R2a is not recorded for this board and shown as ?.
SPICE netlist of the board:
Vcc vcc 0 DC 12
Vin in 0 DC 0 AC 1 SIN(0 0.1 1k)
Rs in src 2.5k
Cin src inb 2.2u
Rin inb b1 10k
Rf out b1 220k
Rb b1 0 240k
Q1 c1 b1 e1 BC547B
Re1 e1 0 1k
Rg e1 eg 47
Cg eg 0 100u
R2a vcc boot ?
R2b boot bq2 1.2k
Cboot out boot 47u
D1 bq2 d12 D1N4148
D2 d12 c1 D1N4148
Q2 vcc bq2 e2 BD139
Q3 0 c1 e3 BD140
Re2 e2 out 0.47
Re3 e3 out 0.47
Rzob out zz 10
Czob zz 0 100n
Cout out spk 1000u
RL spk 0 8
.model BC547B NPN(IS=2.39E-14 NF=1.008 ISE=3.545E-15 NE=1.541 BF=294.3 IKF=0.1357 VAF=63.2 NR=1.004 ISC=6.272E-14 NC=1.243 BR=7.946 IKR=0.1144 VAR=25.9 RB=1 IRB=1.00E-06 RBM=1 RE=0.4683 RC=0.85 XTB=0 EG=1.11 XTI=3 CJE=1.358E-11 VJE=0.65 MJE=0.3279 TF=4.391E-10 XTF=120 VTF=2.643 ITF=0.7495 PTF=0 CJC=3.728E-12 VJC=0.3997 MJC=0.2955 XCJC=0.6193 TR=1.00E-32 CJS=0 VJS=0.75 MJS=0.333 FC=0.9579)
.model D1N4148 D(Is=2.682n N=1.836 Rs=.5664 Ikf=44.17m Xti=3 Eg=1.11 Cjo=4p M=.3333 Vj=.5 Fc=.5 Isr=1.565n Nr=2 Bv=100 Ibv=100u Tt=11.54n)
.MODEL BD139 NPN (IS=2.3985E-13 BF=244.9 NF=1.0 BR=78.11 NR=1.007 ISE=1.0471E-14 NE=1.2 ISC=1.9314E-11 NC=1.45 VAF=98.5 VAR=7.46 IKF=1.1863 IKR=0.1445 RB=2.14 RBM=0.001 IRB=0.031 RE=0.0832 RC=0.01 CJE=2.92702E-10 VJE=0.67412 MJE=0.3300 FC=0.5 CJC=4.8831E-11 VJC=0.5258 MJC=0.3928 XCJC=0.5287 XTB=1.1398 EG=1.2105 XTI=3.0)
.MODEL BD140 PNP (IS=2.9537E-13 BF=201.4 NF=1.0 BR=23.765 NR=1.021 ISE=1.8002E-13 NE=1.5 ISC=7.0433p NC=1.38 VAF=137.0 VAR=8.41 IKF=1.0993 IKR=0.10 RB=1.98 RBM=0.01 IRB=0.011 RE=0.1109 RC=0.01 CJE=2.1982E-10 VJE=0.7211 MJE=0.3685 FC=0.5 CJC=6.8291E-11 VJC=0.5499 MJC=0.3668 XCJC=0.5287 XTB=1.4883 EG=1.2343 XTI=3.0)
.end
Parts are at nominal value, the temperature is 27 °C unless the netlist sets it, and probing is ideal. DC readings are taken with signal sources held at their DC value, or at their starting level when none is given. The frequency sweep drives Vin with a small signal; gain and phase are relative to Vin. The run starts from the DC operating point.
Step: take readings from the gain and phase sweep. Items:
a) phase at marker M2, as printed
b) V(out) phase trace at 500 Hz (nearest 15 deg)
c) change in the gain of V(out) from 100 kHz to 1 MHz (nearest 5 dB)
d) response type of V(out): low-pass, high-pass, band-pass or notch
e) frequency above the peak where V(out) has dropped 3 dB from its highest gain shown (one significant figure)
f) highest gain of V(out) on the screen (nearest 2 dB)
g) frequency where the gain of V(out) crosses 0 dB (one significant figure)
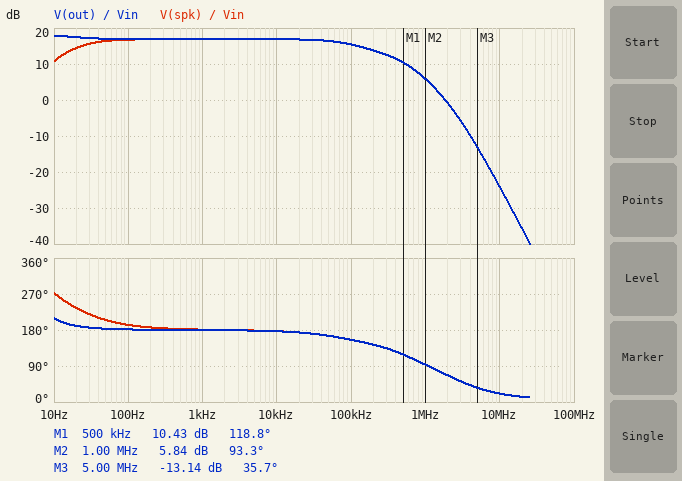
93.3 deg
180 deg
-10 dB
low-pass
100 kHz
18 dB
2 MHz
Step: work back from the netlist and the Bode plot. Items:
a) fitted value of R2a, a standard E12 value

1.2 kΩ
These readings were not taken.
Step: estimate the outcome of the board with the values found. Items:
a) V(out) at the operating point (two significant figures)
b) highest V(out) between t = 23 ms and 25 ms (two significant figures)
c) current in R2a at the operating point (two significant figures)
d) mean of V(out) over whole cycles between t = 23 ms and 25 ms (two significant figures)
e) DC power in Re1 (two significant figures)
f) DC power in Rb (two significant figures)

6.6 V
7.3 V
2.0 mA
6.6 V
4.0 mW
29 µW
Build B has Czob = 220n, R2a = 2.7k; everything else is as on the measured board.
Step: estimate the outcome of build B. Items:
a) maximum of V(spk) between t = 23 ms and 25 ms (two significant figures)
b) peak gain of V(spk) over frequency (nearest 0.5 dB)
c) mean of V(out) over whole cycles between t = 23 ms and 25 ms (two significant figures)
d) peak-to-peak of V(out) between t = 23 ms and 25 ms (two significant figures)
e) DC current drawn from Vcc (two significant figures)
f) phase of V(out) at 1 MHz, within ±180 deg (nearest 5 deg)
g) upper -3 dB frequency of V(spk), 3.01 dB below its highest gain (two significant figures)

680 mV
16.5 dB
5.4 V
1.3 V
10 mA
85 deg
110 kHz
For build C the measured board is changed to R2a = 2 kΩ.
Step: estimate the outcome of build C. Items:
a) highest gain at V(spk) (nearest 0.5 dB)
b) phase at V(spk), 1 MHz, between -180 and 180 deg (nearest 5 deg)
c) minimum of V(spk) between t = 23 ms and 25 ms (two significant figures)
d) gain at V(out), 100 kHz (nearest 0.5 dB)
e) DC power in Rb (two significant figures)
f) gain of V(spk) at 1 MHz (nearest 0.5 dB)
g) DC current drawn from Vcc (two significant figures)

16.5 dB
90 deg
-670 mV
15.0 dB
24 µW
5.0 dB
12 mA
